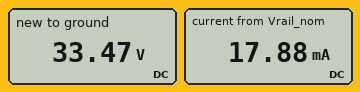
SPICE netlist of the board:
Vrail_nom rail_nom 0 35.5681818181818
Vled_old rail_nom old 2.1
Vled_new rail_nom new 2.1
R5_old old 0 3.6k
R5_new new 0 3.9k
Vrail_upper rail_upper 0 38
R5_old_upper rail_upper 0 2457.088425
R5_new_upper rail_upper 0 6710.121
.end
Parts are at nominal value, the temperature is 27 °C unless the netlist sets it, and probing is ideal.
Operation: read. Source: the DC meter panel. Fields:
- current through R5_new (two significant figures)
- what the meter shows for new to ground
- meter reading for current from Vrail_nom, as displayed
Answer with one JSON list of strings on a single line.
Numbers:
["8.6 mA", "33.47 V", "17.88 mA"]
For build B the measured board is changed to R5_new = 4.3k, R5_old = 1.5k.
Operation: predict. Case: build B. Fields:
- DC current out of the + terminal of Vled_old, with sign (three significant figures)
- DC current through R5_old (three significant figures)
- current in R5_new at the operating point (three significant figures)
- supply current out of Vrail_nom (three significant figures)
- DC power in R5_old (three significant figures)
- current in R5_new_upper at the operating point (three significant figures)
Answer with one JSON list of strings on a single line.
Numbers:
["-22.3 mA", "22.3 mA", "7.78 mA", "30.1 mA", "747 mW", "5.66 mA"]
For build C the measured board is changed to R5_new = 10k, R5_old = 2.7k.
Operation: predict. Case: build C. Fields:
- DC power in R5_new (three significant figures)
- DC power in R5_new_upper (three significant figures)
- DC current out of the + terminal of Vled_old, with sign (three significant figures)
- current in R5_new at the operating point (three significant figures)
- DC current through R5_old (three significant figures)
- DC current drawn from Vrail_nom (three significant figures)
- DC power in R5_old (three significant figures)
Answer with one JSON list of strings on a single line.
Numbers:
["112 mW", "215 mW", "-12.4 mA", "3.35 mA", "12.4 mA", "15.7 mA", "415 mW"]
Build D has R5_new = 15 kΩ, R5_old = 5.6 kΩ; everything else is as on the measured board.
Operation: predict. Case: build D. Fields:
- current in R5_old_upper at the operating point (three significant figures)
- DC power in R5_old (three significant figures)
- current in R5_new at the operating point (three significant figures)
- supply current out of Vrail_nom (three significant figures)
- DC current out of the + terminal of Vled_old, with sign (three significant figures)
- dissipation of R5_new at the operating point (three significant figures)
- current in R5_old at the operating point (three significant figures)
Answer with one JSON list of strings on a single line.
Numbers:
["15.5 mA", "200 mW", "2.23 mA", "8.21 mA", "-5.98 mA", "74.7 mW", "5.98 mA"]
